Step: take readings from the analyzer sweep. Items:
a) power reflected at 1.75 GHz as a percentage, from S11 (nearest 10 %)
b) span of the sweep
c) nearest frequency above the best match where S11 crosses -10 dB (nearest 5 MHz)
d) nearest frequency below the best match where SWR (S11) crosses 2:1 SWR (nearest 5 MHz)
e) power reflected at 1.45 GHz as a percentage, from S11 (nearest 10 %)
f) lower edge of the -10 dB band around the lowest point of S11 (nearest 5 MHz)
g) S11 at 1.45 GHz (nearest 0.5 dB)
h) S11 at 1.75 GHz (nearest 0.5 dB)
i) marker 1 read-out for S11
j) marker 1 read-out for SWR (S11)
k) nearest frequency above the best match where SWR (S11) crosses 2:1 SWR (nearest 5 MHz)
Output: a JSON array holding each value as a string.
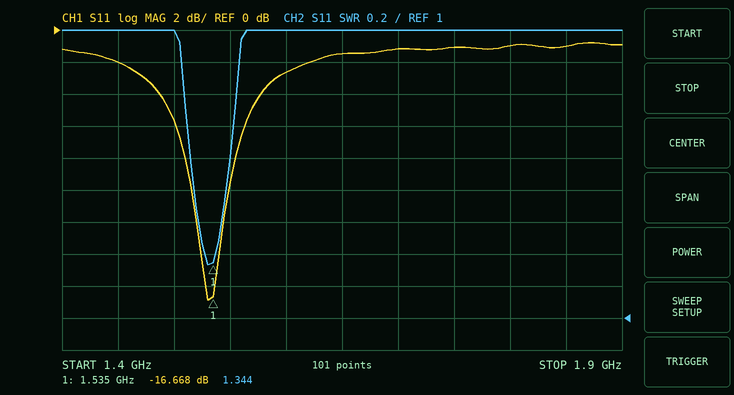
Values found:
["80 %", "500 MHz", "1.550 GHz", "1.515 GHz", "60 %", "1.515 GHz", "-2.0 dB", "-1.0 dB", "-16.668 dB", "1.344", "1.550 GHz"]
